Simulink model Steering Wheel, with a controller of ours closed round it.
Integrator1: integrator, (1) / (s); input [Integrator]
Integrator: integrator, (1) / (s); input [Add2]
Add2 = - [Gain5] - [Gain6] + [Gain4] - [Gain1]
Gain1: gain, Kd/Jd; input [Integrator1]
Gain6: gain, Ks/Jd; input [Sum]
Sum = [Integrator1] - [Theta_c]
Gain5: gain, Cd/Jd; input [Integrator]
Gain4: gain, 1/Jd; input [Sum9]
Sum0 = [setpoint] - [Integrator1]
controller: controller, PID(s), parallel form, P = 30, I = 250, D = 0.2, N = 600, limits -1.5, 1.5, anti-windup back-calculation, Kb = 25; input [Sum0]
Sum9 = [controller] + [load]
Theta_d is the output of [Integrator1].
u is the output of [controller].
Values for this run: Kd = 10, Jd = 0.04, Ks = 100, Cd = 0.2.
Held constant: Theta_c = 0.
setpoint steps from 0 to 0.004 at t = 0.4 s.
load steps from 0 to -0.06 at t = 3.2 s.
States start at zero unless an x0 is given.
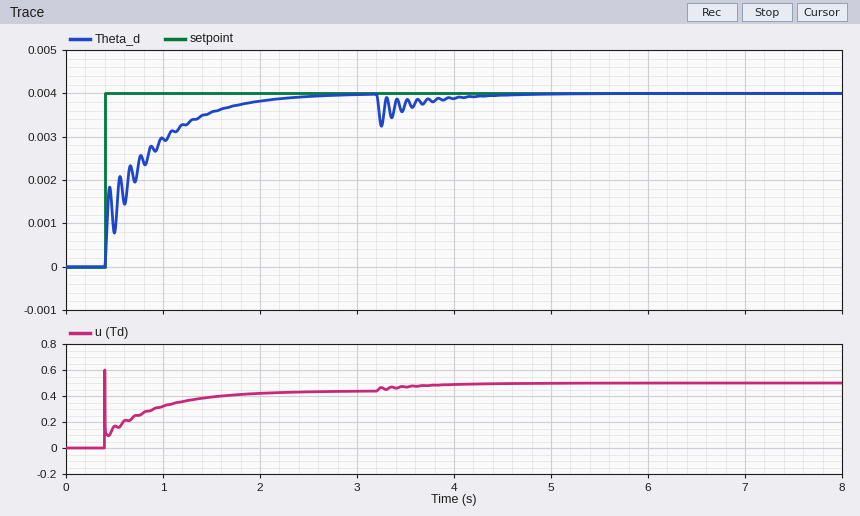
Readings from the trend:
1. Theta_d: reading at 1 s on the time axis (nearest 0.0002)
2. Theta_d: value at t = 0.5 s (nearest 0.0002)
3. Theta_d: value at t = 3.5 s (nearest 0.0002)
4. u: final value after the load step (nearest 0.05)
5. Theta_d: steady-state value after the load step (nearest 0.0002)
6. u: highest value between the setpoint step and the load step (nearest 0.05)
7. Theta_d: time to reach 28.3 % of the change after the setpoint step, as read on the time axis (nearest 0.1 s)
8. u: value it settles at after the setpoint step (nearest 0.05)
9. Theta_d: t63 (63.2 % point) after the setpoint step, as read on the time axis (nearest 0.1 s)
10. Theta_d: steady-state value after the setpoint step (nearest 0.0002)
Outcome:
0.0030
0.0008
0.0038
0.50
0.0040
0.60
0.4 s
0.45
0.8 s
0.0040
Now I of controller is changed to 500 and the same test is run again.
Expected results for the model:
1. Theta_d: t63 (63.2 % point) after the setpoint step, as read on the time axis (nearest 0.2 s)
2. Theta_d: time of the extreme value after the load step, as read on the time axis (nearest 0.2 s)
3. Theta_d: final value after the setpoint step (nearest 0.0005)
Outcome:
0.6 s
3.2 s
0.0040
